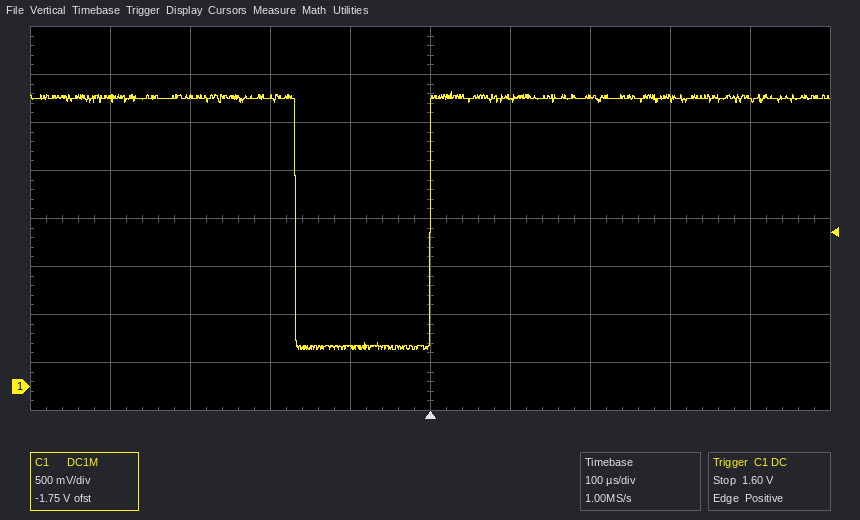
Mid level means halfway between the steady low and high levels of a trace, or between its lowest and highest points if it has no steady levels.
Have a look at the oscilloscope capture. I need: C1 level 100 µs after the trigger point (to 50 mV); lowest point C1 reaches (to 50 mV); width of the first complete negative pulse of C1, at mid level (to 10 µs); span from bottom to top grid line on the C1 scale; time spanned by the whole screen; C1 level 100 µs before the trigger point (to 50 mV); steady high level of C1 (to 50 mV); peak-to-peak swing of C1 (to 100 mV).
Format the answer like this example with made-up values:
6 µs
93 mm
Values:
3.00 V
400 mV
170 µs
4 V
1 ms
400 mV
3.00 V
2.70 V
